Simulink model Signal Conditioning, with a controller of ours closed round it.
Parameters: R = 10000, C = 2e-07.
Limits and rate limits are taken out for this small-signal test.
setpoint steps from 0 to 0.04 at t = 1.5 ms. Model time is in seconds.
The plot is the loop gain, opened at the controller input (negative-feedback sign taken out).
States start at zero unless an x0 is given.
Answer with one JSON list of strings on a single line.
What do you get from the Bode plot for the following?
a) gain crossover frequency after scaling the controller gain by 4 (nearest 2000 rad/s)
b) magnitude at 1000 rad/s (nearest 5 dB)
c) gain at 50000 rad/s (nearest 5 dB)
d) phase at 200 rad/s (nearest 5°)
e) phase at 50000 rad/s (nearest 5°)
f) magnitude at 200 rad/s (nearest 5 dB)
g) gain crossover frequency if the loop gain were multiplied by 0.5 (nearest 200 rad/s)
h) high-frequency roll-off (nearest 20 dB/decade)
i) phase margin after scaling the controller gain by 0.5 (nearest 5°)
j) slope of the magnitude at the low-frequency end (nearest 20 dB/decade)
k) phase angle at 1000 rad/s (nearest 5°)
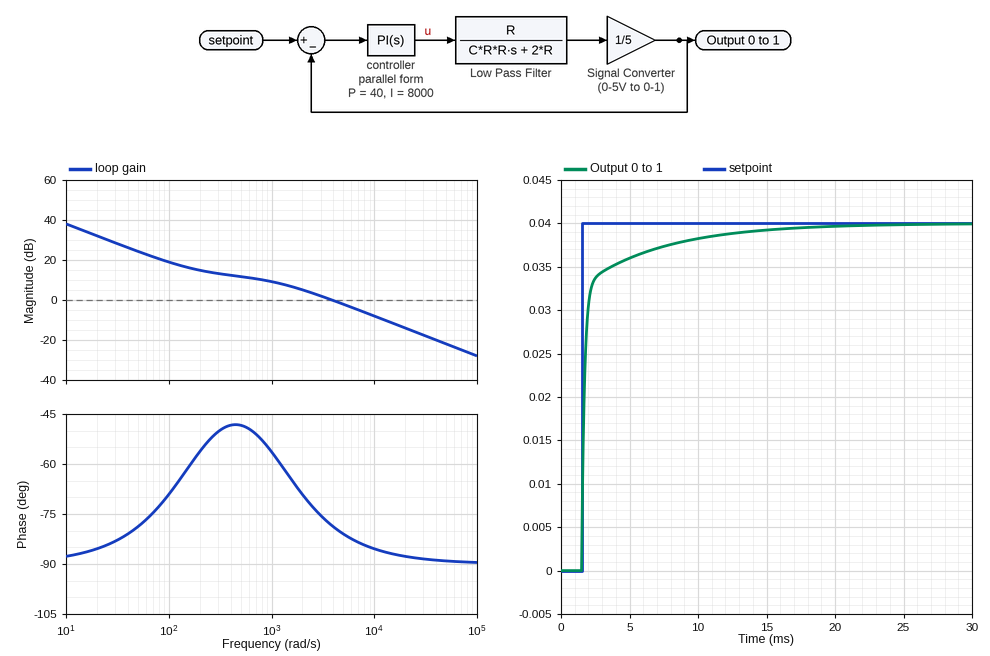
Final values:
["16000 rad/s", "10 dB", "-20 dB", "-55°", "-90°", "15 dB", "1800 rad/s", "-20 dB/decade", "115°", "-20 dB/decade", "-55°"]
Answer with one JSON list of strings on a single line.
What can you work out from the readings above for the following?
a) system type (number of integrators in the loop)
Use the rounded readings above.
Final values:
["1"]
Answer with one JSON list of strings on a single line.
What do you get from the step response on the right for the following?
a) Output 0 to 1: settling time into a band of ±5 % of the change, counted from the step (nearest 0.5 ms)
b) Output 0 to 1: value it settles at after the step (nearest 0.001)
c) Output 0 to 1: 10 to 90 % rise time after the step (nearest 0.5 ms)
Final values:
["7.5 ms", "0.040", "3.5 ms"]
